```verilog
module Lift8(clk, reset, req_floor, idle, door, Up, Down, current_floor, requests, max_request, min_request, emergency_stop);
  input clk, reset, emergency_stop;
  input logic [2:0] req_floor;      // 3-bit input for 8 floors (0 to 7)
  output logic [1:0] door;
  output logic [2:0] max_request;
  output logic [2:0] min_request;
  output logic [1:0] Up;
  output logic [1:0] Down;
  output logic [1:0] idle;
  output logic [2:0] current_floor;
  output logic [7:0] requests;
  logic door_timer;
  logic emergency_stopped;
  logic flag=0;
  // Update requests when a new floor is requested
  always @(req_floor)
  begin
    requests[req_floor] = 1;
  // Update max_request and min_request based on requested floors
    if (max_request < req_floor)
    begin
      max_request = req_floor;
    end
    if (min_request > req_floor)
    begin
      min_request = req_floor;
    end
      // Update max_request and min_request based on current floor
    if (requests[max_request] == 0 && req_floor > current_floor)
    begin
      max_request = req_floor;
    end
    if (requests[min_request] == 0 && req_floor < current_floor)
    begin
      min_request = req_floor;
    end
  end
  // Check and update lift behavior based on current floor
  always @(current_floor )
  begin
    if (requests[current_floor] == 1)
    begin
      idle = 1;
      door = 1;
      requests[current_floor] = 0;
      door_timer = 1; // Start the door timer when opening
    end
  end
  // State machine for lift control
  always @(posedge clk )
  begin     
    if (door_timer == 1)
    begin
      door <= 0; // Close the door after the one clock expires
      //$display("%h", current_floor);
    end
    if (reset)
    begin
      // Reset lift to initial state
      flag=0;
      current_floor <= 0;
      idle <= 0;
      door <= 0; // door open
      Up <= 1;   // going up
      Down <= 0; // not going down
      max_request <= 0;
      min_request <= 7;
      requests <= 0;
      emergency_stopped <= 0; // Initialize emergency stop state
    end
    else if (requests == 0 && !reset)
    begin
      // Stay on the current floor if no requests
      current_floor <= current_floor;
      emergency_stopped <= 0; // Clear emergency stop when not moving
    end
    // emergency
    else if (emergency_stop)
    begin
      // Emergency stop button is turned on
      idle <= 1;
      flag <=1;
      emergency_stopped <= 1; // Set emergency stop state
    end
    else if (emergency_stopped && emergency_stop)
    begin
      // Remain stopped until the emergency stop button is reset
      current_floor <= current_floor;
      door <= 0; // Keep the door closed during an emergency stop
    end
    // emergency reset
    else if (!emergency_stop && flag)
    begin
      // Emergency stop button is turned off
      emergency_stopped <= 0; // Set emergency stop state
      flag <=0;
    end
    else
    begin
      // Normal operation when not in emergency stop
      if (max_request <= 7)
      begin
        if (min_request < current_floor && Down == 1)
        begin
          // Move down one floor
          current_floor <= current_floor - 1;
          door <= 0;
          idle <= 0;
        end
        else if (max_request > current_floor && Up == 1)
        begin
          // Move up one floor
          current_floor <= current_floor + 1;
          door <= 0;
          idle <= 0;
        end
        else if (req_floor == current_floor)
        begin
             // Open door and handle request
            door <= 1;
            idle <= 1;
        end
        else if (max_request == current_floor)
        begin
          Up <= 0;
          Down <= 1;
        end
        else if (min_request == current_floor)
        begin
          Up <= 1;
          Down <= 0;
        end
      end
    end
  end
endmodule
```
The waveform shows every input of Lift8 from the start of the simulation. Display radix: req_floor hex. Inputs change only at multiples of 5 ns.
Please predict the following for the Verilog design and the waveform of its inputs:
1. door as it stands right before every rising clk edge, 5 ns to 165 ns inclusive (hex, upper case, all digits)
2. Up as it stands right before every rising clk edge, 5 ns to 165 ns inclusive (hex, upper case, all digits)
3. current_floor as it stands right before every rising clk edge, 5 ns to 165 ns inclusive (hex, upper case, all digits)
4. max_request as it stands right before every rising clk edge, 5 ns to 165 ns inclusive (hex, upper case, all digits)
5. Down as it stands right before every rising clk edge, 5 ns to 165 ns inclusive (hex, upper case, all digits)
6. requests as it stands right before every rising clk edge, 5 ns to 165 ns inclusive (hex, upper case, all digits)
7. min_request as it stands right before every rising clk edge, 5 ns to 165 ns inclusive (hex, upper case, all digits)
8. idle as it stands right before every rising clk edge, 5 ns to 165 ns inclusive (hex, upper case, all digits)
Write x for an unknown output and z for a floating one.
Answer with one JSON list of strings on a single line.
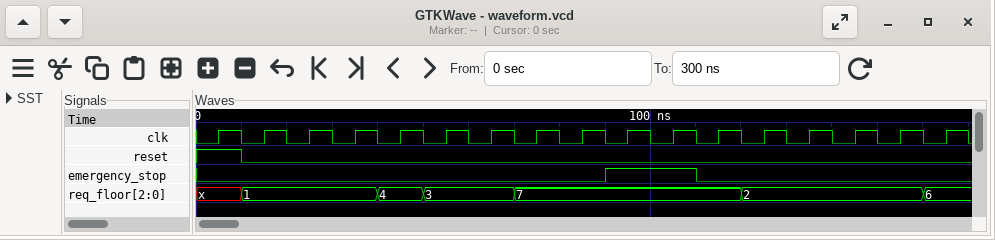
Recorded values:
["x, 0, 1, 0, 0, 0, 1, 1, 0, 0, 0, 0, 0, 1, 0, 0, 0", "x, 1, 1, 1, 1, 1, 1, 1, 1, 1, 1, 1, 1, 1, 0, 0, 0", "x, 0, 1, 1, 1, 2, 3, 4, 5, 6, 6, 6, 6, 7, 7, 6, 5", "x, 1, 1, 1, 4, 4, 4, 7, 7, 7, 7, 7, 7, 7, 7, 7, 6", "x, 0, 0, 0, 0, 0, 0, 0, 0, 0, 0, 0, 0, 0, 1, 1, 1", "x, 02, 00, 00, 10, 18, 10, 80, 80, 80, 80, 80, 84, 04, 04, 04, 44", "x, 1, 1, 1, 1, 1, 1, 1, 1, 1, 1, 1, 2, 2, 2, 2, 2", "x, 0, 1, 1, 1, 0, 1, 1, 0, 0, 1, 1, 1, 1, 1, 0, 0"]
